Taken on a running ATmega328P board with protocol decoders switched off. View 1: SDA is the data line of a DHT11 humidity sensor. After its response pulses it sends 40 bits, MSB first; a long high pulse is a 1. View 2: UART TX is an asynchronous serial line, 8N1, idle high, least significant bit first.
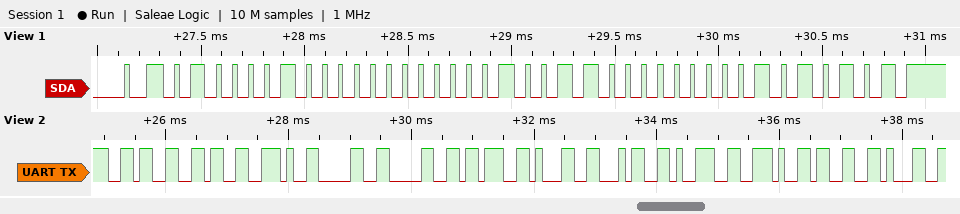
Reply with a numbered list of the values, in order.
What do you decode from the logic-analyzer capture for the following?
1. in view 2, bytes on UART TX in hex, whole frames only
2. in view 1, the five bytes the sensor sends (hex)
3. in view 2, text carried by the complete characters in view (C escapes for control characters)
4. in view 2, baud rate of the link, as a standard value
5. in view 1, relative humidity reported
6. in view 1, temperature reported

1. 36 36 2E 30 30 3B 31 34 39 2E 33 31
2. 42 00 13 00 55
3. "66.00;149.31"
4. 9600 baud
5. 66 %
6. 19.0 °C
